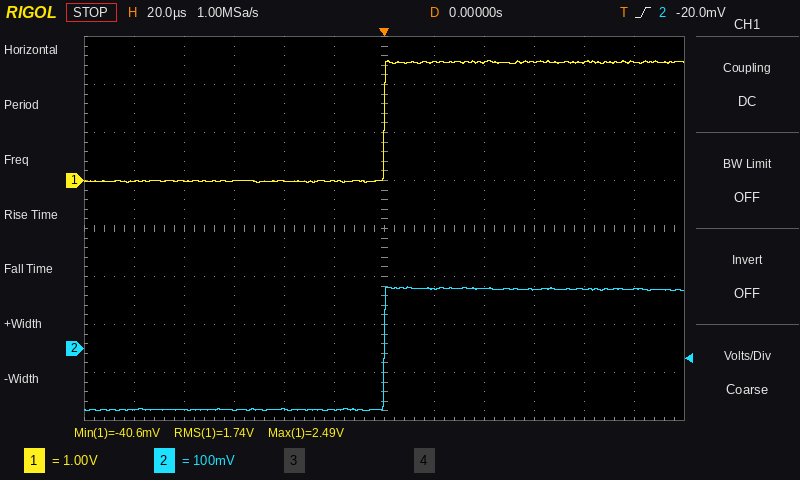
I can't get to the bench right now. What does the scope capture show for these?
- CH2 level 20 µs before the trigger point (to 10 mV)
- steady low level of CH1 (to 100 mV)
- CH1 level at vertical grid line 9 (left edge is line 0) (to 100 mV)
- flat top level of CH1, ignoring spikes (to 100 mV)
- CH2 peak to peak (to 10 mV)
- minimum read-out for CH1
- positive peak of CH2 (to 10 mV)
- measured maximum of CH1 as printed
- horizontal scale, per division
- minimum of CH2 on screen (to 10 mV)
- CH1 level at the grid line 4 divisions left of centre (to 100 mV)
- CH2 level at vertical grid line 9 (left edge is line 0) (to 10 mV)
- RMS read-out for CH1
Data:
-130 mV
0.0 V
2.5 V
2.5 V
260 mV
-40.6 mV
130 mV
2.49 V
20 µs
-130 mV
0.0 V
120 mV
1.74 V
